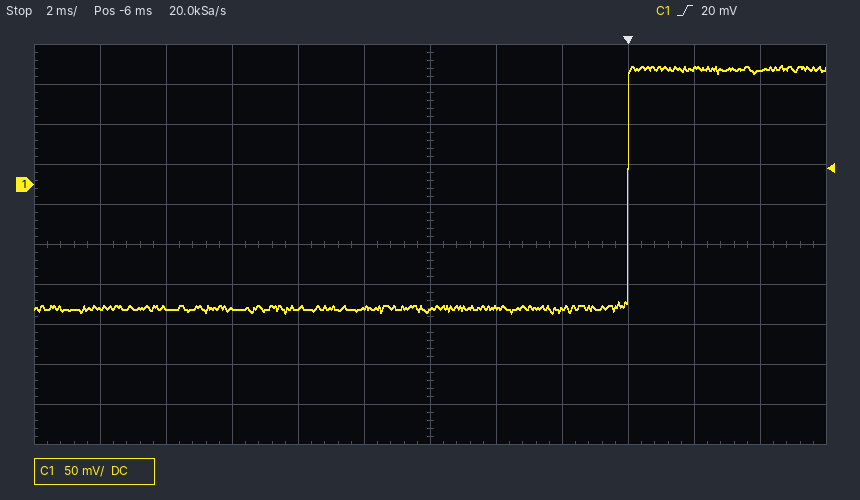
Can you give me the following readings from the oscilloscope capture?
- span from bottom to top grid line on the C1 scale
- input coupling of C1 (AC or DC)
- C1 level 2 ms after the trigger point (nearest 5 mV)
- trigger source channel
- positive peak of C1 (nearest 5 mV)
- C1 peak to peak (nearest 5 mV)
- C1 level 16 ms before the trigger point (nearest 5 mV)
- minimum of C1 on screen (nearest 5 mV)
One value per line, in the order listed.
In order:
500 mV
DC
145 mV
C1
150 mV
310 mV
-155 mV
-160 mV
